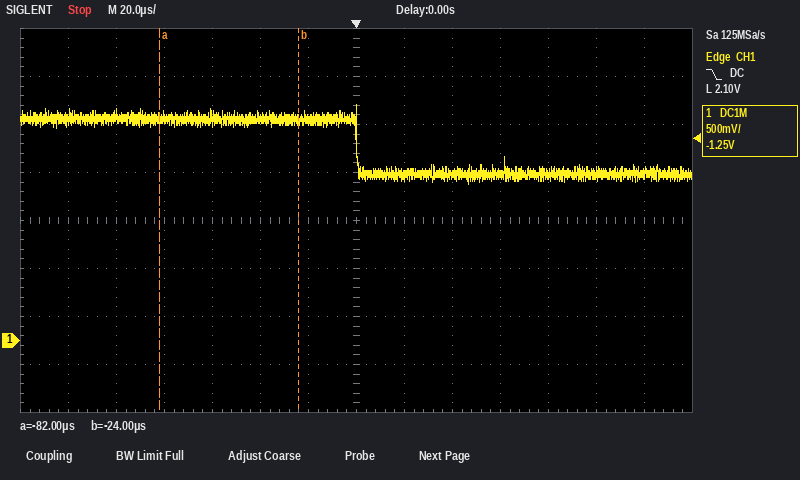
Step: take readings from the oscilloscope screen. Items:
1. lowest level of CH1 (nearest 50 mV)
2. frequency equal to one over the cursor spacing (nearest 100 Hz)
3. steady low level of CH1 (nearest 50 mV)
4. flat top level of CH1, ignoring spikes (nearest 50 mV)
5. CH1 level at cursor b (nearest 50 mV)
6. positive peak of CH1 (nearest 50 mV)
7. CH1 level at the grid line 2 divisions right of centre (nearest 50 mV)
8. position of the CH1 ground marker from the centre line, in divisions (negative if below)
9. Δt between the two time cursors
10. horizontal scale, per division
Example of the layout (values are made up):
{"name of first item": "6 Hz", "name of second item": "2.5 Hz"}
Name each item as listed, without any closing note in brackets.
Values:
{"lowest level of CH1": "1.65 V", "frequency equal to one over the cursor spacing": "17.2 kHz", "steady low level of CH1": "1.75 V", "flat top level of CH1, ignoring spikes": "2.30 V", "CH1 level at cursor b": "2.30 V", "positive peak of CH1": "2.45 V", "CH1 level at the grid line 2 divisions right of centre": "1.75 V", "position of the CH1 ground marker from the centre line, in divisions": "-2.5 div", "Δt between the two time cursors": "58 µs", "horizontal scale, per division": "20 µs"}
